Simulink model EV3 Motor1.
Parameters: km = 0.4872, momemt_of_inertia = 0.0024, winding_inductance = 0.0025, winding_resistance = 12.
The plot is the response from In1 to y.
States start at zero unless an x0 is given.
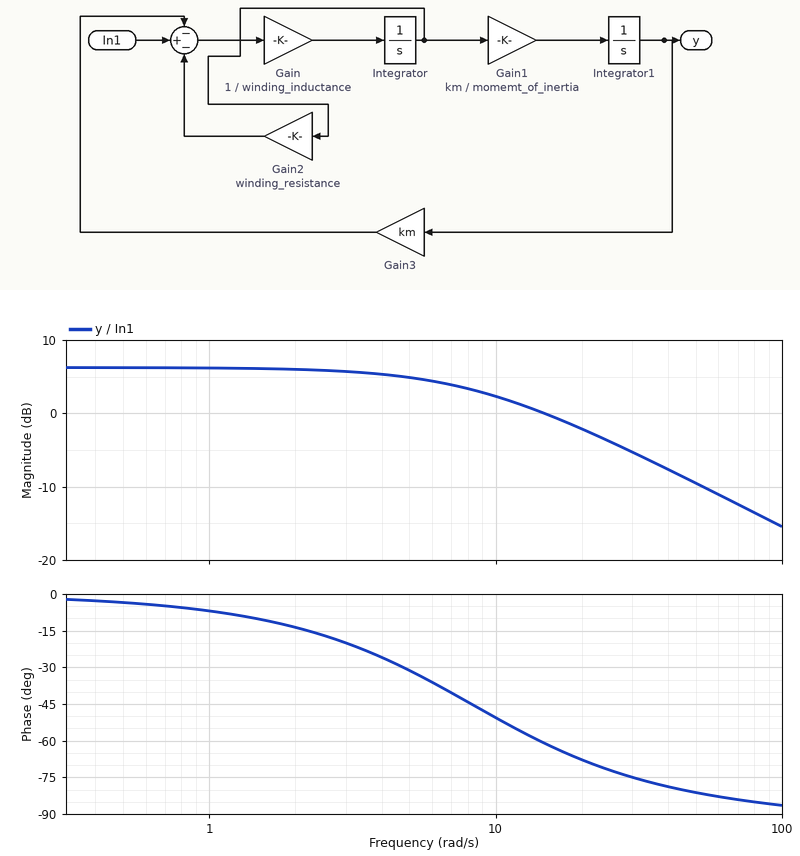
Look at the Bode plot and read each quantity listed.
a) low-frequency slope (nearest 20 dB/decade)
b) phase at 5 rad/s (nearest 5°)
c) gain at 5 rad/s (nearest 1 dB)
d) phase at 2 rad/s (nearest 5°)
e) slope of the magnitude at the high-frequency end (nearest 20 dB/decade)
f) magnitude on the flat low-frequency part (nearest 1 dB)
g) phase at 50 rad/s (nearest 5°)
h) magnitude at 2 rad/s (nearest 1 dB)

0 dB/decade
-30°
5 dB
-15°
-20 dB/decade
6 dB
-80°
6 dB
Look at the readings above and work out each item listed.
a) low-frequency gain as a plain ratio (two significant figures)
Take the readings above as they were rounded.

2.0
